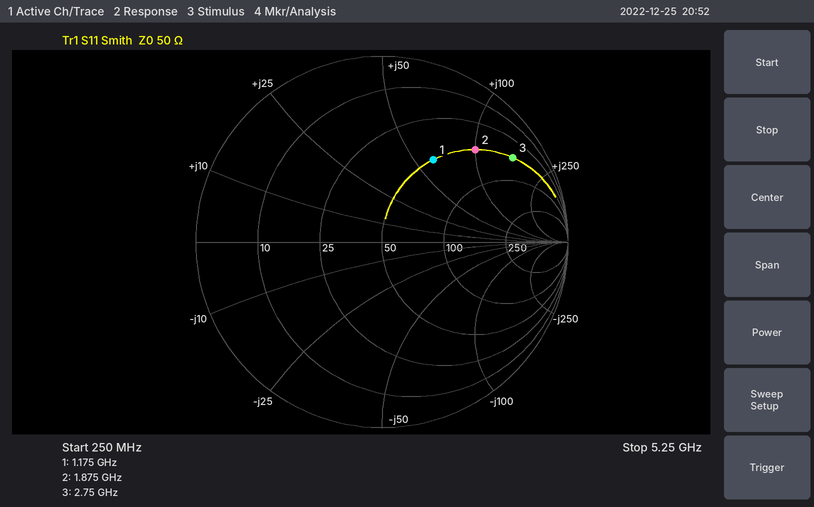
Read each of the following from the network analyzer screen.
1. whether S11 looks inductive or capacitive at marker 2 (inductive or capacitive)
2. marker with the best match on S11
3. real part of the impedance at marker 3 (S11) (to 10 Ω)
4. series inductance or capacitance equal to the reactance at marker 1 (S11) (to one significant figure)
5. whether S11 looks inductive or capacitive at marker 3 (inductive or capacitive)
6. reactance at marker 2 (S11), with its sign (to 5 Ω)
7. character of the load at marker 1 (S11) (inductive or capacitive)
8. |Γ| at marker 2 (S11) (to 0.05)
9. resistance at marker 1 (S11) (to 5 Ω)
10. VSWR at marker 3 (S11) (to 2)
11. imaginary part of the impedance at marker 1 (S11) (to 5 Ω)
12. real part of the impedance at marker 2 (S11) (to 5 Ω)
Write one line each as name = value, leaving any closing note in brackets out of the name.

whether S11 looks inductive or capacitive at marker 2 = inductive
marker with the best match on S11 = marker 1
real part of the impedance at marker 3 (S11) = 50 Ω
series inductance or capacitance equal to the reactance at marker 1 (S11) = 8 nH
whether S11 looks inductive or capacitive at marker 3 = inductive
reactance at marker 2 (S11), with its sign = +100 Ω
character of the load at marker 1 (S11) = inductive
|Γ| at marker 2 (S11) = 0.70
resistance at marker 1 (S11) = 50 Ω
VSWR at marker 3 (S11) = 12
imaginary part of the impedance at marker 1 (S11) = +60 Ω
real part of the impedance at marker 2 (S11) = 50 Ω
